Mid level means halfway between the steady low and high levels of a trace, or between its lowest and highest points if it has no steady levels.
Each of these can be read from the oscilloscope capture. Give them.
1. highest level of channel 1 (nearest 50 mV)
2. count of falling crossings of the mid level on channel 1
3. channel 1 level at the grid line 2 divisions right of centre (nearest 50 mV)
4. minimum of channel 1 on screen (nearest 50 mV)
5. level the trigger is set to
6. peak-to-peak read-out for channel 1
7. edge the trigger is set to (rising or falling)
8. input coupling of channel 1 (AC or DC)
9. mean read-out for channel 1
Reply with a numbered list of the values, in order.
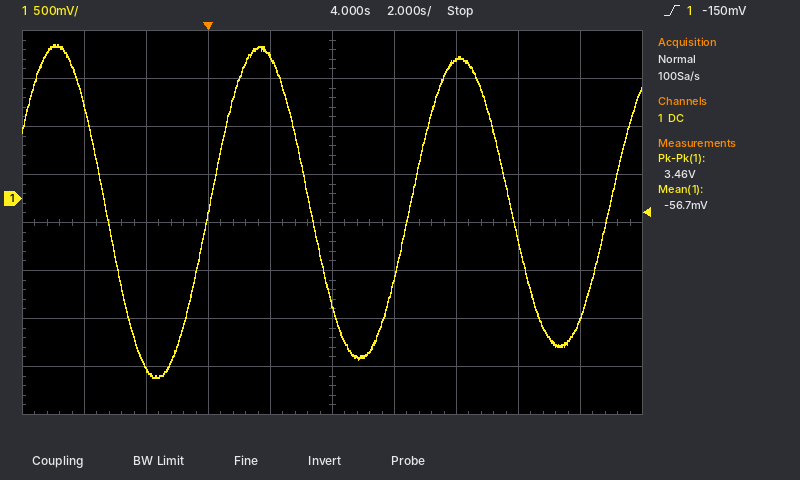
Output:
1. 1.60 V
2. 3
3. 1.45 V
4. -1.85 V
5. -150 mV
6. 3.46 V
7. rising
8. DC
9. -56.7 mV
